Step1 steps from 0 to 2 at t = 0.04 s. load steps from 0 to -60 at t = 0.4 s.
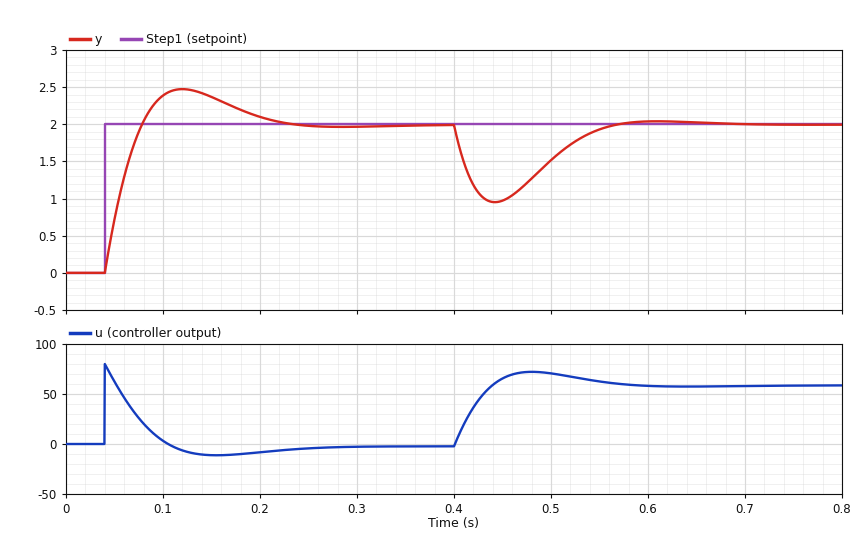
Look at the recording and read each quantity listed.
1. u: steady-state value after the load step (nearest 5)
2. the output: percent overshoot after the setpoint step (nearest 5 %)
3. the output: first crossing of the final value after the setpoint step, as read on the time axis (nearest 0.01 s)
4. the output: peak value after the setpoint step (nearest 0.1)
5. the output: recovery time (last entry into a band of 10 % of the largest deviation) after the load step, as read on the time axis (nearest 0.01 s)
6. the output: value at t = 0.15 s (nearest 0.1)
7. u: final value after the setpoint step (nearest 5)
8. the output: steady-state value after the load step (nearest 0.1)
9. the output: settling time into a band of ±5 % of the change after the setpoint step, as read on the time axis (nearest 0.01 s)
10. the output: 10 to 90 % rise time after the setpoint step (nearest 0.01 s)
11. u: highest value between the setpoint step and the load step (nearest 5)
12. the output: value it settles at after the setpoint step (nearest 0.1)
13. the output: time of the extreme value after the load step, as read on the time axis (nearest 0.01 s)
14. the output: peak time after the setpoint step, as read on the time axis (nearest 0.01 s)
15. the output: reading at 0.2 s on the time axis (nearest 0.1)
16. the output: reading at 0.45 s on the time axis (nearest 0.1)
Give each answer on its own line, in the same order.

60
25 %
0.08 s
2.5
0.54 s
2.4
0
2.0
0.20 s
0.03 s
80
2.0
0.44 s
0.12 s
2.1
1.0
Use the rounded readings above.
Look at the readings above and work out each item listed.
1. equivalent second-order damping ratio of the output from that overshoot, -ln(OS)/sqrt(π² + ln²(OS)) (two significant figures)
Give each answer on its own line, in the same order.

0.40
